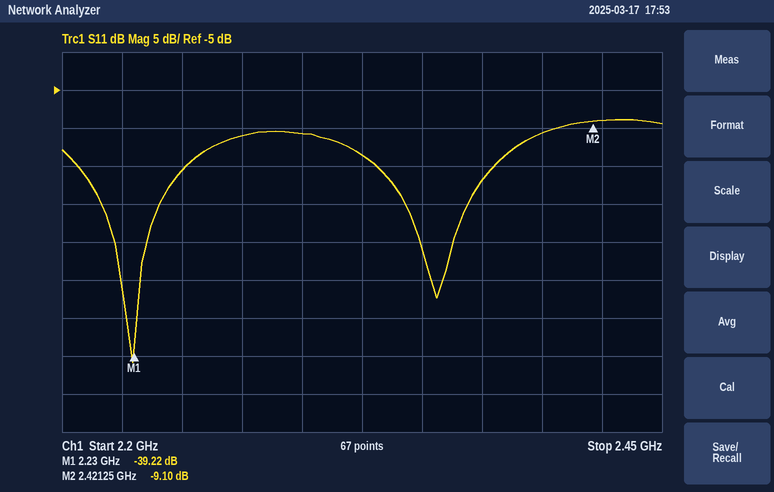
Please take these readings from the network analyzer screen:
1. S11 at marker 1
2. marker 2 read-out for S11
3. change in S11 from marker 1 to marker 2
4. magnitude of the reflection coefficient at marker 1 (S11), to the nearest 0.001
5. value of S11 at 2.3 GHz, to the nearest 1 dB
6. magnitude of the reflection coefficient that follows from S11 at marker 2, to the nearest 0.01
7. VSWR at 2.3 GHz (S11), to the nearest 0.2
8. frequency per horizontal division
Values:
-39.22 dB
-9.10 dB
30.12 dB
0.011
-11 dB
0.35
1.8
25 MHz
